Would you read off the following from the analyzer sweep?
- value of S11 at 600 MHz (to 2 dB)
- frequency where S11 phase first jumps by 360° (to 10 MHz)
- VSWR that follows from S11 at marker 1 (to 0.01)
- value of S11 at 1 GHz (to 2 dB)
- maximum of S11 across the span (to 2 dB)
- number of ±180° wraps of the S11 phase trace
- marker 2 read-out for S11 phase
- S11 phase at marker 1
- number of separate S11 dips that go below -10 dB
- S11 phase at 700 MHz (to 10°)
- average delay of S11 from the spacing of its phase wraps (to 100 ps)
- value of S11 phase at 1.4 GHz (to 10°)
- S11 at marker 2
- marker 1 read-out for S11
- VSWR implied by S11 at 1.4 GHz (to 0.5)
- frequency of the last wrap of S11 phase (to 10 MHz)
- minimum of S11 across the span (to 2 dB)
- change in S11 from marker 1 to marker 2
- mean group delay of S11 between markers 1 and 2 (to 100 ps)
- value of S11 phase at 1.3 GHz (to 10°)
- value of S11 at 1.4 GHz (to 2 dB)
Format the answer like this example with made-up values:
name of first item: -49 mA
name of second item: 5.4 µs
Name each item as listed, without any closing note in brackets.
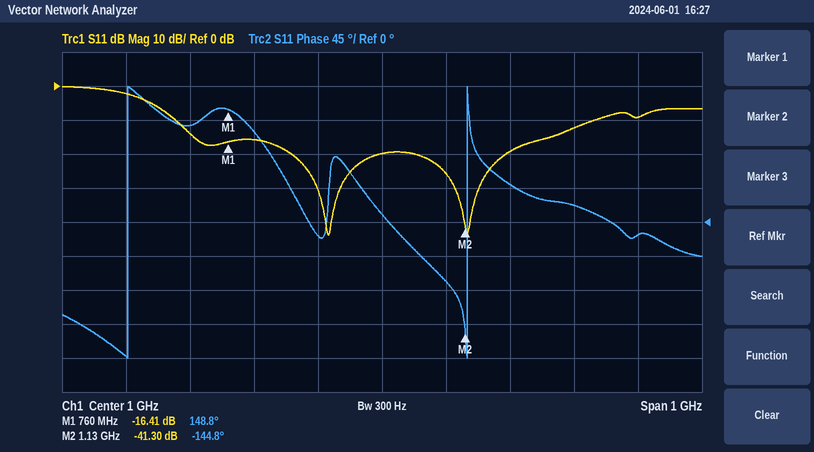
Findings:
value of S11 at 600 MHz: -2 dB
frequency where S11 phase first jumps by 360°: 600 MHz
VSWR that follows from S11 at marker 1: 1.36
value of S11 at 1 GHz: -20 dB
maximum of S11 across the span: 0 dB
number of ±180° wraps of the S11 phase trace: 2
marker 2 read-out for S11 phase: -144.8°
S11 phase at marker 1: 148.8°
number of separate S11 dips that go below -10 dB: 2
S11 phase at 700 MHz: 130°
average delay of S11 from the spacing of its phase wraps: 1.9 ns
value of S11 phase at 1.4 GHz: -20°
S11 at marker 2: -41.30 dB
marker 1 read-out for S11: -16.41 dB
VSWR implied by S11 at 1.4 GHz: 2.0
frequency of the last wrap of S11 phase: 1.13 GHz
minimum of S11 across the span: -44 dB
change in S11 from marker 1 to marker 2: -24.89 dB
mean group delay of S11 between markers 1 and 2: 2.2 ns
value of S11 phase at 1.3 GHz: 20°
value of S11 at 1.4 GHz: -10 dB
